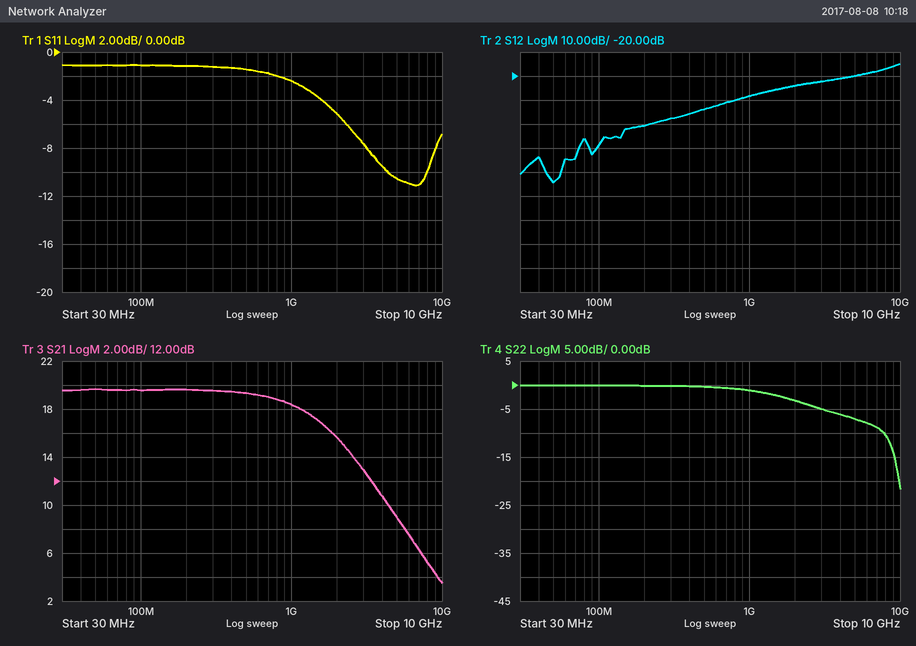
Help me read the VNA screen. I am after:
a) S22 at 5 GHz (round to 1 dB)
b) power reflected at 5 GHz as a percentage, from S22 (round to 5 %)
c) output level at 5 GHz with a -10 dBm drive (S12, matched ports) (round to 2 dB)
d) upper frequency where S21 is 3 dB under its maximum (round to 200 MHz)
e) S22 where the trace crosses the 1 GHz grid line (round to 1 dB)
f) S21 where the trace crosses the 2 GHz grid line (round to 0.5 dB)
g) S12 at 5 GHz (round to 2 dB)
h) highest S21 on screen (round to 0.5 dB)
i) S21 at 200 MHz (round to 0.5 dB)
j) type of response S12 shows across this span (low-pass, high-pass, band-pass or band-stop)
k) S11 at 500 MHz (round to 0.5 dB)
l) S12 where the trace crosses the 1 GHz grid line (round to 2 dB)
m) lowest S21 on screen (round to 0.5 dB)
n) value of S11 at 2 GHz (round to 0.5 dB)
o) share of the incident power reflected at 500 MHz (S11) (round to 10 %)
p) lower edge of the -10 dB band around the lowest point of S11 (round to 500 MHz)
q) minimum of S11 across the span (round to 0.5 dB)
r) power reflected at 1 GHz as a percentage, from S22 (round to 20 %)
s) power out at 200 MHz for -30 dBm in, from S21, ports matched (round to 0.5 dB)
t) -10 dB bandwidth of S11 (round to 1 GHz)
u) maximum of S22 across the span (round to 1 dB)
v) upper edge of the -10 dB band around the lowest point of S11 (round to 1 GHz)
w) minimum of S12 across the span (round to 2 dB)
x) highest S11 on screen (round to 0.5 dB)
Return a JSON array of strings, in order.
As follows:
["-7 dB", "20 %", "-30 dBm", "1.6 GHz", "-1 dB", "15.5 dB", "-20 dB", "19.5 dB", "19.5 dB", "high-pass", "-1.5 dB", "-28 dB", "3.5 dB", "-5.0 dB", "70 %", "4.5 GHz", "-11.0 dB", "80 %", "-10.5 dBm", "4 GHz", "0 dB", "8 GHz", "-64 dB", "-1.0 dB"]
